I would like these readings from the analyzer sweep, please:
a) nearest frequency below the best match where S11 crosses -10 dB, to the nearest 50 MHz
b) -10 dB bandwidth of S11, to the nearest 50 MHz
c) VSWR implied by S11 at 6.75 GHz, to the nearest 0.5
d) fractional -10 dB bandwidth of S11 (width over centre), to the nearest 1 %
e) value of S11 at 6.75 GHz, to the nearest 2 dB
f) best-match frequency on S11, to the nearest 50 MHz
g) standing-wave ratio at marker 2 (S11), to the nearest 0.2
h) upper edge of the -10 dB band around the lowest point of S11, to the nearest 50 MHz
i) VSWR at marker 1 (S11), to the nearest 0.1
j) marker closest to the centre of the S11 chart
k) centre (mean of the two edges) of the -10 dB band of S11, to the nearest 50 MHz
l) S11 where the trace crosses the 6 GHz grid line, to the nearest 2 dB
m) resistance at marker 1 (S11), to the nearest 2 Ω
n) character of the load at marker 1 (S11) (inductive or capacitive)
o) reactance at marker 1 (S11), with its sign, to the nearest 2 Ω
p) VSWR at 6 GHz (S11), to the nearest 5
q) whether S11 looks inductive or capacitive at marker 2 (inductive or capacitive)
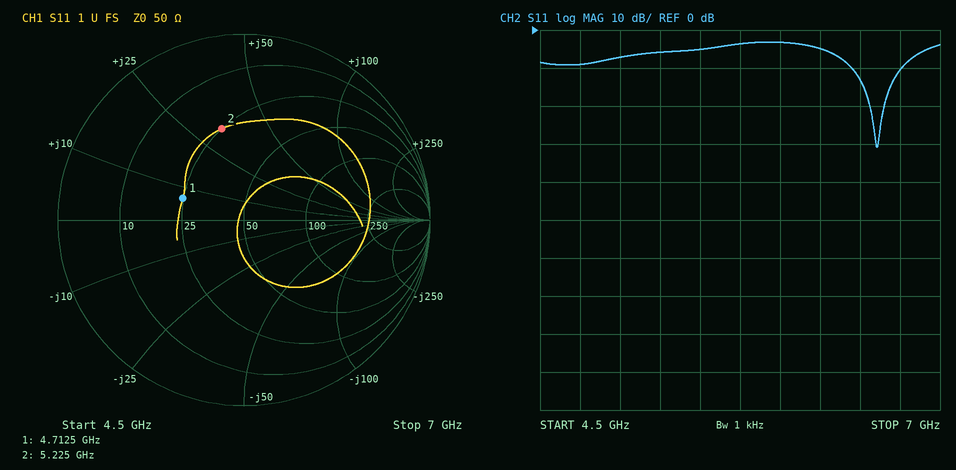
6.45 GHz
300 MHz
2.0
5 %
-10 dB
6.60 GHz
3.0
6.75 GHz
2.1
marker 1
6.60 GHz
-4 dB
24 Ω
inductive
+6 Ω
5
inductive
